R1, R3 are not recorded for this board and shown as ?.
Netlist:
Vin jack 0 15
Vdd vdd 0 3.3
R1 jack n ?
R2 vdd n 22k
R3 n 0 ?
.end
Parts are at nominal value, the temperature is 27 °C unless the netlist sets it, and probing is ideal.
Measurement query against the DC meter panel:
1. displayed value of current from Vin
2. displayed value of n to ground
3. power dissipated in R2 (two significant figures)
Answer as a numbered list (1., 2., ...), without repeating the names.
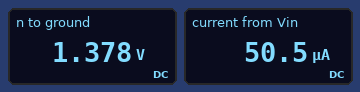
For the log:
1. 50.5 µA
2. 1.378 V
3. 170 µW
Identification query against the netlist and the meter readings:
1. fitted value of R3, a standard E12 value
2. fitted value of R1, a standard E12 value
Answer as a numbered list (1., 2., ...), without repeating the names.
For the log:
1. 10 kΩ
2. 270 kΩ
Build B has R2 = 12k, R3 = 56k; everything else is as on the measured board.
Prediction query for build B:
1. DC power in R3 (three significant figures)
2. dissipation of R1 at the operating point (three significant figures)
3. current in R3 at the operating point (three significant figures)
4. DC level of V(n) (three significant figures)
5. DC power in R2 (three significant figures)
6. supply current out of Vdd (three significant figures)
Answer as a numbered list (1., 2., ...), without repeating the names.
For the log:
1. 177 µW
2. 520 µW
3. 56.3 µA
4. 3.15 V
5. 1.84 µW
6. 12.4 µA
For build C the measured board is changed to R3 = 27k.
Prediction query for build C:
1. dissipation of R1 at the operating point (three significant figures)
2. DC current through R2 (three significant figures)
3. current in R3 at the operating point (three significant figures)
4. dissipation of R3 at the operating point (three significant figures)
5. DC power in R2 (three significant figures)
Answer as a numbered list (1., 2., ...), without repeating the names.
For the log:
1. 589 µW
2. 41.6 µA
3. 88.3 µA
4. 211 µW
5. 38.1 µW
